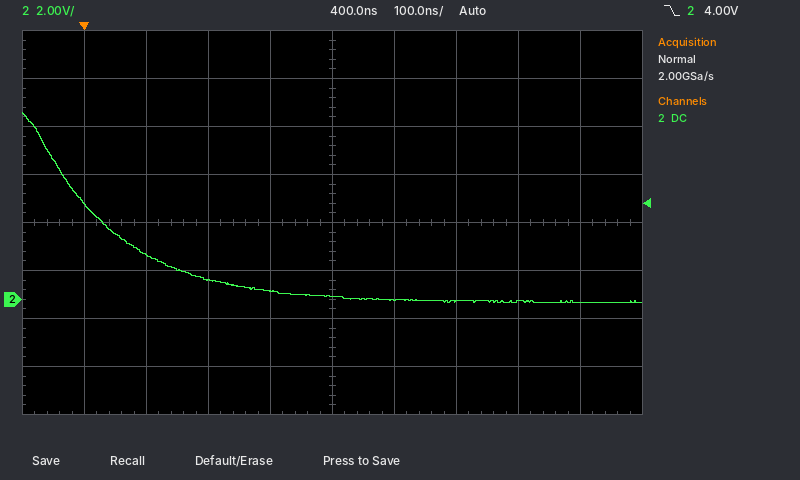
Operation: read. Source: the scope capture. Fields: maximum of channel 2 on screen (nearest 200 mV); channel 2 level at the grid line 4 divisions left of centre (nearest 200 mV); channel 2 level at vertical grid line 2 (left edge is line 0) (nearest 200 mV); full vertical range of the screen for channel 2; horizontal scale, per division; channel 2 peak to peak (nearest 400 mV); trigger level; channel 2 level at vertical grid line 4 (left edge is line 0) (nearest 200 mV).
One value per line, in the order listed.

7.8 V
4.0 V
1.8 V
16 V
100 ns
8.0 V
4.00 V
400 mV
